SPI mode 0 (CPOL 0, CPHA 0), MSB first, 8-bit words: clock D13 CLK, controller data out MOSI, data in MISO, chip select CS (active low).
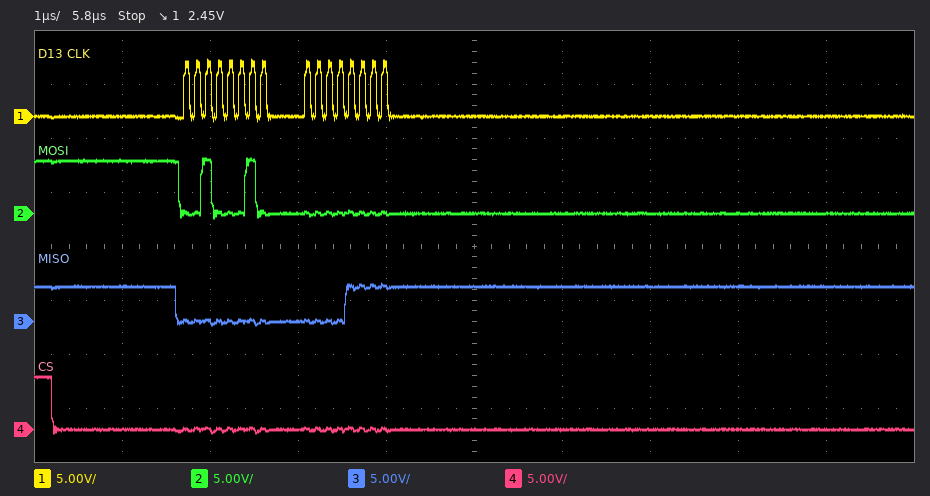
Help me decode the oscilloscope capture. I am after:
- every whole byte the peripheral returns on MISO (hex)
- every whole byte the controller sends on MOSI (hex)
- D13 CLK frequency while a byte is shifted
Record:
00 0F
22 00
8 MHz
